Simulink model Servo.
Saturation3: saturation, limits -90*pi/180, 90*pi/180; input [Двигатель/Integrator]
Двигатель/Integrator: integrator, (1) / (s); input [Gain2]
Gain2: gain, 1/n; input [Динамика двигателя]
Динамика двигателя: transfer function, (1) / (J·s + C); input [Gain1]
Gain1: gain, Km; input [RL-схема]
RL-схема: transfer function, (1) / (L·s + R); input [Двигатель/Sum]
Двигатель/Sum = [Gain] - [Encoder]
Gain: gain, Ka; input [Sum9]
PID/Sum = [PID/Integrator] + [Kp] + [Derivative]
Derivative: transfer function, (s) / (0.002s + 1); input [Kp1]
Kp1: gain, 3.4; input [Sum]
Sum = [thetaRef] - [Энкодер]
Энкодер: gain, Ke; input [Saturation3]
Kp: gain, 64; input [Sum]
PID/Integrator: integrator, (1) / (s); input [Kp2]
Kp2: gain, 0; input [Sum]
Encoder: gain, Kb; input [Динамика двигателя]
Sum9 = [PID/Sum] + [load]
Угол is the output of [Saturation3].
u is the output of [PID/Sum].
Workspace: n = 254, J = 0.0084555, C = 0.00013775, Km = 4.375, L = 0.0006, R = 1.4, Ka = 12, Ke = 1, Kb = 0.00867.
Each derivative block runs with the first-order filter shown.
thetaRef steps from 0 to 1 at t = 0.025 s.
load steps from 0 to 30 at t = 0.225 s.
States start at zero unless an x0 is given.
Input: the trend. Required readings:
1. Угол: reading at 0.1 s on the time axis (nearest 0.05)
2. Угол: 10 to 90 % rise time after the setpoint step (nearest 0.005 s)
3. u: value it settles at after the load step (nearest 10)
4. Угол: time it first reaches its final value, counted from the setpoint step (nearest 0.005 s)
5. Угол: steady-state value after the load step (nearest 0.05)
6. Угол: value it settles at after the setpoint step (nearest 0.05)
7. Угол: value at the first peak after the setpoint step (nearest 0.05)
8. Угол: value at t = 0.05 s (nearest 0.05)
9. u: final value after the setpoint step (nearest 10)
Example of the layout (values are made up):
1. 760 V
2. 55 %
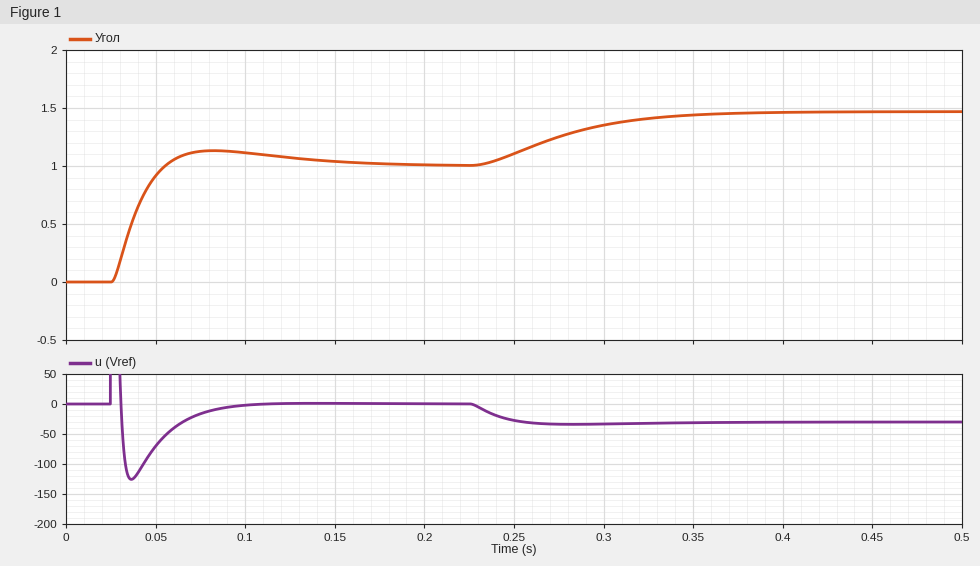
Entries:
1. 1.10
2. 0.020 s
3. -30
4. 0.030 s
5. 1.45
6. 1.00
7. 1.15
8. 0.90
9. 0
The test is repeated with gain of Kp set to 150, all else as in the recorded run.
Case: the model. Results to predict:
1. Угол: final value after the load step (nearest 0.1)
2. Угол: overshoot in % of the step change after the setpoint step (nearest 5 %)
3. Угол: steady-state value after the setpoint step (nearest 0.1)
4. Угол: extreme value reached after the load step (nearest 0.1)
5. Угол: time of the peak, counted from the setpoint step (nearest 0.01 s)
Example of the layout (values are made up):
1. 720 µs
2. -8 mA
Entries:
1. 1.2
2. 25 %
3. 1.0
4. 1.2
5. 0.04 s
